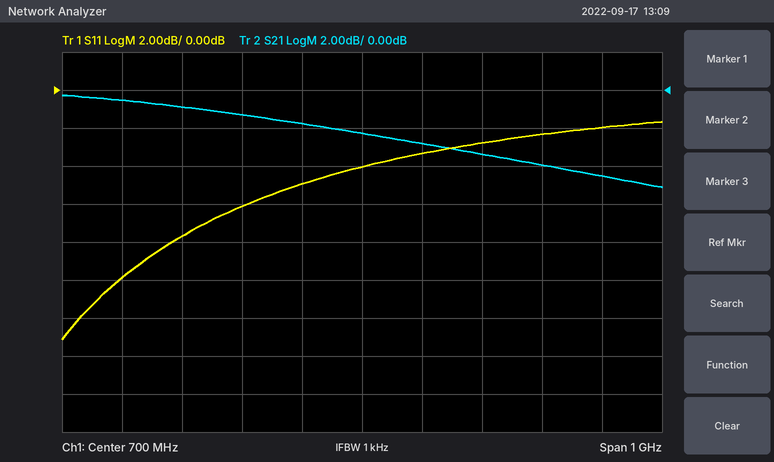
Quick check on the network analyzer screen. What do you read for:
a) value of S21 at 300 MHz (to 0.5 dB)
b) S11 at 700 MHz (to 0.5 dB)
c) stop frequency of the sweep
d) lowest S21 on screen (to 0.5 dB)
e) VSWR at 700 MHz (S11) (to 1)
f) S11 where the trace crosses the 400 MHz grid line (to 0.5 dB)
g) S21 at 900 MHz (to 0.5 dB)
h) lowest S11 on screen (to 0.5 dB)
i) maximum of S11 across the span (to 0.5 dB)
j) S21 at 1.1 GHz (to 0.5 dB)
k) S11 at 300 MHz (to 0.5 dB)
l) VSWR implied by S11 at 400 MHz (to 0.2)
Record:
-0.5 dB
-4.0 dB
1.2 GHz
-5.0 dB
4
-7.5 dB
-3.5 dB
-13.0 dB
-1.5 dB
-4.5 dB
-10.0 dB
2.4
